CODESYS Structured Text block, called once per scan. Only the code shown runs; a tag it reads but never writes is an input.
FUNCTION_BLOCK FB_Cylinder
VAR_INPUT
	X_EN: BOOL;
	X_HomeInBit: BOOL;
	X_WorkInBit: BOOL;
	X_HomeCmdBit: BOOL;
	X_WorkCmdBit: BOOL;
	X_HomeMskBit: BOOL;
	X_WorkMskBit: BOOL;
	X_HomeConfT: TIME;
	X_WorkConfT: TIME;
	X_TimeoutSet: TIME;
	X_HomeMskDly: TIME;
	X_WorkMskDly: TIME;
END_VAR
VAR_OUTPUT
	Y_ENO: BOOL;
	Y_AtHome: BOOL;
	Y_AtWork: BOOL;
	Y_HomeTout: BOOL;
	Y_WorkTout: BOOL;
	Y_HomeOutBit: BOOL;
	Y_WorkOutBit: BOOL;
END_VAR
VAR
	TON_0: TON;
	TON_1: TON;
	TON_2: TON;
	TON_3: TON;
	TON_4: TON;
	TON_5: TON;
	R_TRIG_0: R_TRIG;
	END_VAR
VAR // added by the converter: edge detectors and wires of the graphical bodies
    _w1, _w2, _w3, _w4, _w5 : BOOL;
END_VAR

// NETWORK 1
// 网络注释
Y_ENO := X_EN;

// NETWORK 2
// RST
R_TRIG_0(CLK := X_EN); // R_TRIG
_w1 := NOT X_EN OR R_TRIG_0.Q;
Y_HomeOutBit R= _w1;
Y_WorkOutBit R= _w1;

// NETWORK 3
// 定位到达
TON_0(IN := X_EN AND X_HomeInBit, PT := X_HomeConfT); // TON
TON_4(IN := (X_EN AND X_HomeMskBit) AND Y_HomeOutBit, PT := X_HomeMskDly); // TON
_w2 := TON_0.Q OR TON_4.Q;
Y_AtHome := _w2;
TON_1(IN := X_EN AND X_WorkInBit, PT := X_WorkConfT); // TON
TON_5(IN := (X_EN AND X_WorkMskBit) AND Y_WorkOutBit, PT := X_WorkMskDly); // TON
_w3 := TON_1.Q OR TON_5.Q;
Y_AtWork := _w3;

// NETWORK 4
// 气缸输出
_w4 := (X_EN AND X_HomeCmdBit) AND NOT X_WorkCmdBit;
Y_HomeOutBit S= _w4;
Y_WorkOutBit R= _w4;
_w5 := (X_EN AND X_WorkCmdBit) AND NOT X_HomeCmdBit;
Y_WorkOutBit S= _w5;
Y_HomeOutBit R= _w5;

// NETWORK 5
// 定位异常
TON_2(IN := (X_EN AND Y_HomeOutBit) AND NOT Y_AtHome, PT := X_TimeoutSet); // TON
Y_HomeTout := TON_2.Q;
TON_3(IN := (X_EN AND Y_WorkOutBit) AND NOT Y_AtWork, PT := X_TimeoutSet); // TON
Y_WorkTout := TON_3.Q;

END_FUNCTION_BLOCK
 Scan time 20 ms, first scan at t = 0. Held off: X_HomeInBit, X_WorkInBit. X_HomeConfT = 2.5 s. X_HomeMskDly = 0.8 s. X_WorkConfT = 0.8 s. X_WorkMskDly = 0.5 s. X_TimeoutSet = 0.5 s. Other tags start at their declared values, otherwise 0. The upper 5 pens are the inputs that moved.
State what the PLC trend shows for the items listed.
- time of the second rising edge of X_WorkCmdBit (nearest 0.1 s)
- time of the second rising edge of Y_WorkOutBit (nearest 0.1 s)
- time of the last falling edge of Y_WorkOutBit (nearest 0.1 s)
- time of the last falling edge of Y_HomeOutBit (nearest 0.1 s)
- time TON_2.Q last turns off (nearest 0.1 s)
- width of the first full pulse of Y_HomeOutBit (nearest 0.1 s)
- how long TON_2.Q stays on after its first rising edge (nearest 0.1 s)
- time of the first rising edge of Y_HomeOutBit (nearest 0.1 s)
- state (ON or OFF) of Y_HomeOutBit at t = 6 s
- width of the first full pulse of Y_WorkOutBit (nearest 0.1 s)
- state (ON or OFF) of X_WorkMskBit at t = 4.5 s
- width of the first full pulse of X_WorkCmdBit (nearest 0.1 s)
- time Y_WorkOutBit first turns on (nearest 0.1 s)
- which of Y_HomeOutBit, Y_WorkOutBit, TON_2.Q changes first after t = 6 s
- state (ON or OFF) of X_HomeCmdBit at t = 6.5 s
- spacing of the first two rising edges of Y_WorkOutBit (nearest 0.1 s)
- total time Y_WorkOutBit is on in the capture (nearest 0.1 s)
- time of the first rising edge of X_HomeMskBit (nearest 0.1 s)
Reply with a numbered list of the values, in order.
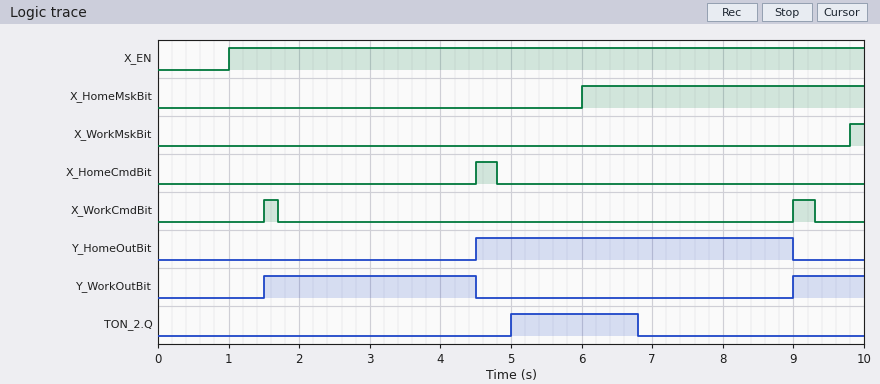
1. 9.0 s
2. 9.0 s
3. 4.5 s
4. 9.0 s
5. 6.8 s
6. 4.5 s
7. 1.8 s
8. 4.5 s
9. ON
10. 3.0 s
11. OFF
12. 0.2 s
13. 1.5 s
14. TON_2.Q
15. OFF
16. 7.5 s
17. 4.0 s
18. 6.0 s
